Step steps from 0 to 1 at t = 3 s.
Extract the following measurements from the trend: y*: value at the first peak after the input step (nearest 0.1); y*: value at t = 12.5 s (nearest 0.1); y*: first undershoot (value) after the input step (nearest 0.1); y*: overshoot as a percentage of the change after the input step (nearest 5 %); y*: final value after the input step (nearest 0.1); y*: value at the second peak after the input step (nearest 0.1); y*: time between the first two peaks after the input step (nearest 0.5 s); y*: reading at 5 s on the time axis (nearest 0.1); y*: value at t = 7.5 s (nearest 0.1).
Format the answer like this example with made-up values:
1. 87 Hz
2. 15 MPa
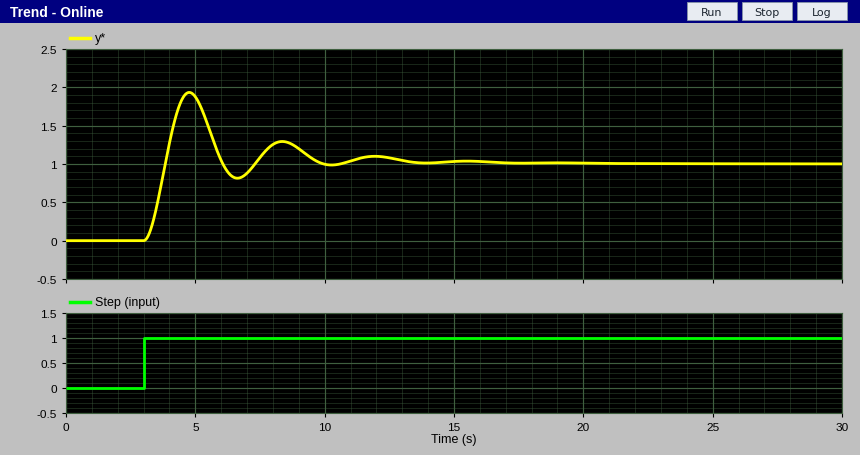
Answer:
1. 1.9
2. 1.1
3. 0.8
4. 95 %
5. 1.0
6. 1.3
7. 3.5 s
8. 1.9
9. 1.1
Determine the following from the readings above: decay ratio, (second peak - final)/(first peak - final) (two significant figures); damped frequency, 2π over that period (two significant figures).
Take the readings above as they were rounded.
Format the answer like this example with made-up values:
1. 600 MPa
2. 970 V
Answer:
1. 0.33
2. 1.8 rad/s
